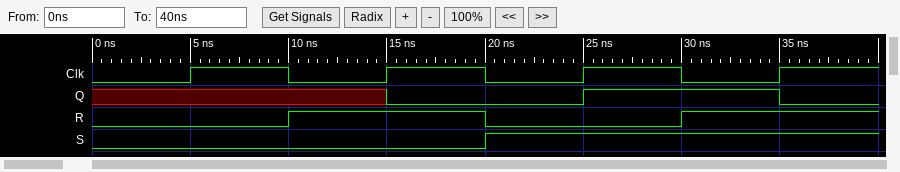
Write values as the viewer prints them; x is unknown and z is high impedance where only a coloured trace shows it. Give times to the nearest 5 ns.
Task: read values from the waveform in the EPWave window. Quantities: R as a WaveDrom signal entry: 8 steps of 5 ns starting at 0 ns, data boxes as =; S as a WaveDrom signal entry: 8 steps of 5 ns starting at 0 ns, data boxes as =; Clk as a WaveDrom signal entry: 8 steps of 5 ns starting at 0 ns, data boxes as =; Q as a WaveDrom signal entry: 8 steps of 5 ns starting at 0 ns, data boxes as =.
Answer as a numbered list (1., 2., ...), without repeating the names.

1. {name: 'R', wave: '0.1.0.1.'}
2. {name: 'S', wave: '0...1...'}
3. {name: 'Clk', wave: '01010101'}
4. {name: 'Q', wave: 'x..0.1.0'}
